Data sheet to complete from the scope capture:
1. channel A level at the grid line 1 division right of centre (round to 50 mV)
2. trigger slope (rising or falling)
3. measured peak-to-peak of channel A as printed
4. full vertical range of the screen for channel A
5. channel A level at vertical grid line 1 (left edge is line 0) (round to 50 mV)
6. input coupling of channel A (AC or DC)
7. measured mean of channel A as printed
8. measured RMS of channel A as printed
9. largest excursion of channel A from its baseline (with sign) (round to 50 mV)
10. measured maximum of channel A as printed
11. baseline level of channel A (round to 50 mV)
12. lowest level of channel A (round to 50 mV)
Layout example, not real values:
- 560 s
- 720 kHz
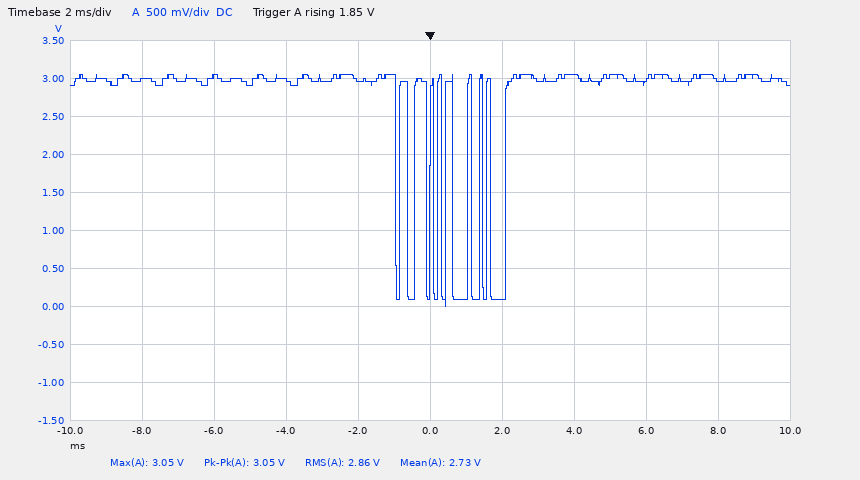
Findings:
- 100 mV
- rising
- 3.05 V
- 5 V
- 3.00 V
- DC
- 2.73 V
- 2.86 V
- -3.00 V
- 3.05 V
- 3.00 V
- 0 mV
